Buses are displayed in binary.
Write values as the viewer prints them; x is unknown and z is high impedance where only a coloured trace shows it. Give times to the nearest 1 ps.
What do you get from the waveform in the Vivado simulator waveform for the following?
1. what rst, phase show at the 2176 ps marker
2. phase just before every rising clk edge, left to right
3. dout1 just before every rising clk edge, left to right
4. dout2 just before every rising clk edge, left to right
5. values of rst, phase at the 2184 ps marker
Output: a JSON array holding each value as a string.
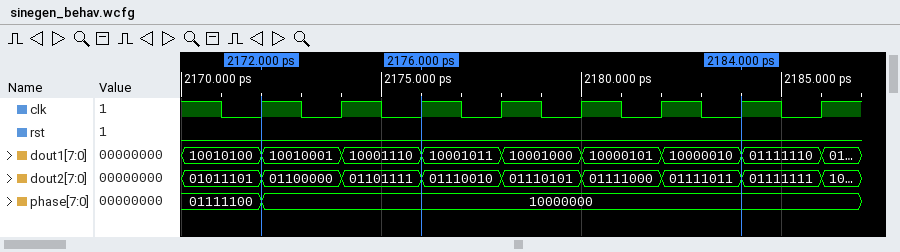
["rst=0, phase=10000000", "01111100, 10000000, 10000000, 10000000, 10000000, 10000000, 10000000, 10000000", "10010100, 10010001, 10001110, 10001011, 10001000, 10000101, 10000010, 01111110", "01011101, 01100000, 01101111, 01110010, 01110101, 01111000, 01111011, 01111111", "rst=0, phase=10000000"]
